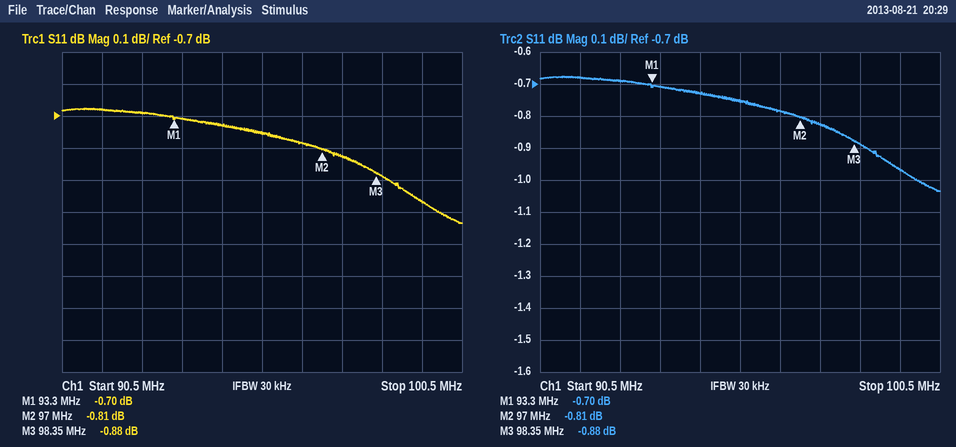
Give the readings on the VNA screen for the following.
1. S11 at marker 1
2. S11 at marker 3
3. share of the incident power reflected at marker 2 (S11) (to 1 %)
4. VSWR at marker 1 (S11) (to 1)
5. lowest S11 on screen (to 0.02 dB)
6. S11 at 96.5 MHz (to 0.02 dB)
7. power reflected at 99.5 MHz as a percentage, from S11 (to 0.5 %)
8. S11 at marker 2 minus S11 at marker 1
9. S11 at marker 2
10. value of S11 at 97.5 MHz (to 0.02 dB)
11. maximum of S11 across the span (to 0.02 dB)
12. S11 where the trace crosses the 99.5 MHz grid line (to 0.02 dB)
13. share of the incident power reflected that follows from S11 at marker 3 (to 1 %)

-0.70 dB
-0.88 dB
83 %
25
-1.04 dB
-0.78 dB
80.0 %
-0.11 dB
-0.81 dB
-0.82 dB
-0.68 dB
-0.96 dB
82 %
